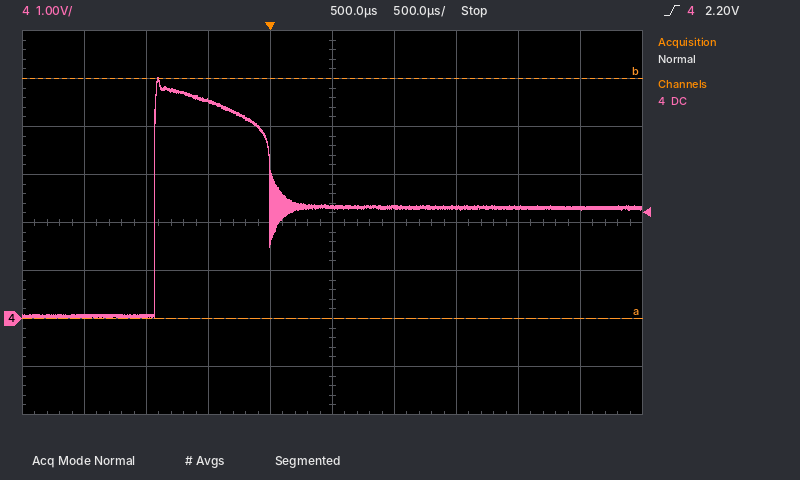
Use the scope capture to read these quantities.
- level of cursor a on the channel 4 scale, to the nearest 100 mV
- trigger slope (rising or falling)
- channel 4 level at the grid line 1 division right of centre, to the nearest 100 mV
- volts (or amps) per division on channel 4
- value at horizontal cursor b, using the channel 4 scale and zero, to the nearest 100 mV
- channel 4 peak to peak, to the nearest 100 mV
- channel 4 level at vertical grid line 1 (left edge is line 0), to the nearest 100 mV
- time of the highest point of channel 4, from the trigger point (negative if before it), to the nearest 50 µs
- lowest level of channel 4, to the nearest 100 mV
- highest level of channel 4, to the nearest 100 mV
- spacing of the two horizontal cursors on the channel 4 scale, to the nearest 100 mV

0.0 V
rising
2.3 V
1 V
5.0 V
5.0 V
100 mV
-900 µs
0.0 V
5.0 V
5.0 V
